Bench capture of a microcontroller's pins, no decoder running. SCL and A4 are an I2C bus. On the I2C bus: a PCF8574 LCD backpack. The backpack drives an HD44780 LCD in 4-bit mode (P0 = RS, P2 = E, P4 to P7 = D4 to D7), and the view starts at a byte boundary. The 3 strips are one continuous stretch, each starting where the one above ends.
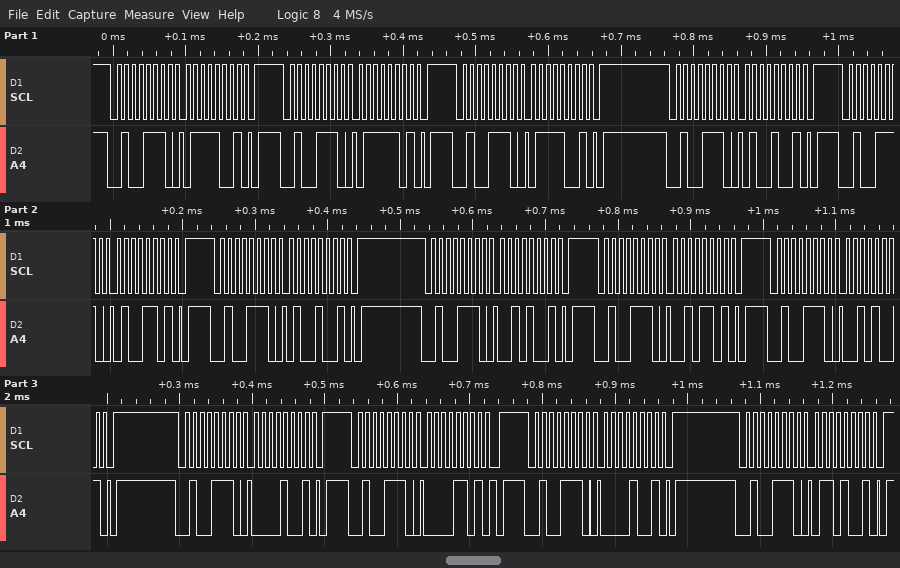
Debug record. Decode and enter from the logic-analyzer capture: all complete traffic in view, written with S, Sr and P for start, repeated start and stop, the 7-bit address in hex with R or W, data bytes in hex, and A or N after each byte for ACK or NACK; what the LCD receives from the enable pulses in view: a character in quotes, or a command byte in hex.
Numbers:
S 27W A 79 A P S 27W A 7D A P S 27W A 79 A P S 27W A 49 A P S 27W A 4D A P S 27W A 49 A P S 27W A 29 A P S 27W A 2D A P S 27W A 29 A P S 27W A 09 A P S 27W A 0D A P S 27W A 09 A P S 27W A 69 A P
't' ' '
